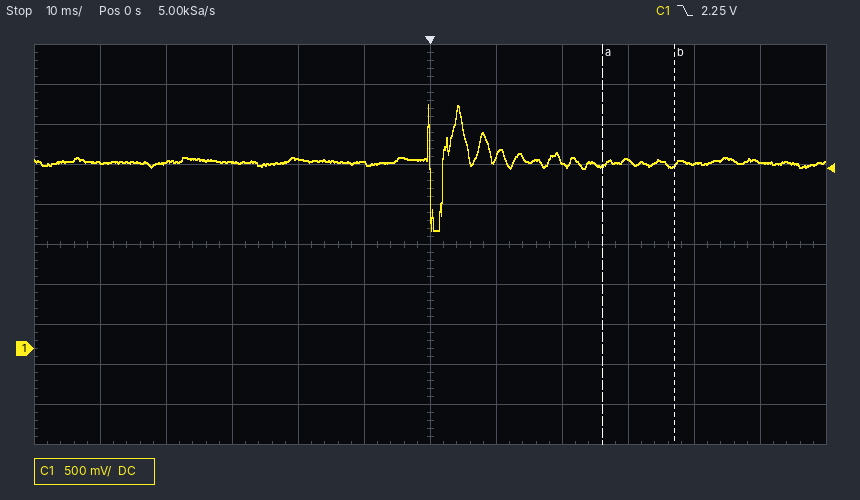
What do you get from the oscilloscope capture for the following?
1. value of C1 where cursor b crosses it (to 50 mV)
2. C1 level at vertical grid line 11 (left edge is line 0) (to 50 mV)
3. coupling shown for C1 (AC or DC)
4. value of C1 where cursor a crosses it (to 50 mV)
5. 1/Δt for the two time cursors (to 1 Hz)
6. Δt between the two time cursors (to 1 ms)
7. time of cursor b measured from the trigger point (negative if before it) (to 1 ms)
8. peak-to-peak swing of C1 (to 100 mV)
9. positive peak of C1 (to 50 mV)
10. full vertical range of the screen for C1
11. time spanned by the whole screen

2.30 V
2.35 V
DC
2.30 V
91 Hz
11 ms
+37 ms
1.60 V
3.05 V
5 V
120 ms
